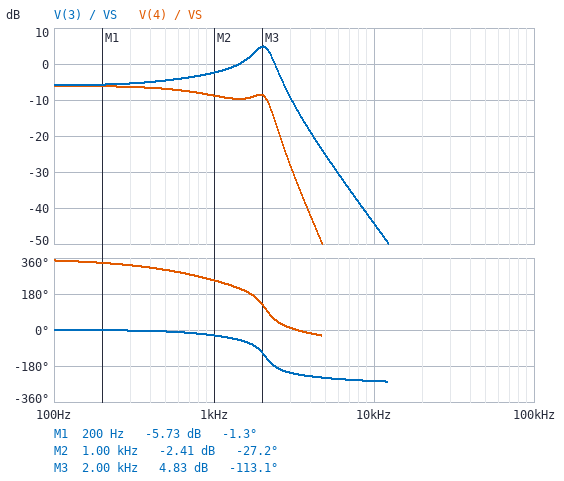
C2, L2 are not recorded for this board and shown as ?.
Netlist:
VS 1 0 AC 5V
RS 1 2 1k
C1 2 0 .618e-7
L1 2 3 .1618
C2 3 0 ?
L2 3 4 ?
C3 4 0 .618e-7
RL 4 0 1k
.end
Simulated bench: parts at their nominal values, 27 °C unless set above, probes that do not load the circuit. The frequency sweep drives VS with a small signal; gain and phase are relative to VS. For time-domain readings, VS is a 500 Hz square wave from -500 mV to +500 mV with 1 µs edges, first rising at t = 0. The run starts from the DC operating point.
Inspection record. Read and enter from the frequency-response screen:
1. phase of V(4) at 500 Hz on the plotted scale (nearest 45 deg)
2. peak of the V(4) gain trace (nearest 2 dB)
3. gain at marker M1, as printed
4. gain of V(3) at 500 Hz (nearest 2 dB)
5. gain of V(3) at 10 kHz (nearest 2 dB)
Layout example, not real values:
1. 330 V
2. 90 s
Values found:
1. 315 deg
2. -6 dB
3. -5.73 dB
4. -4 dB
5. -44 dB
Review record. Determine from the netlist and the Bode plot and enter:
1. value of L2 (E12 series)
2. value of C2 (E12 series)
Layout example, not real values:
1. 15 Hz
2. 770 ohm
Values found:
1. 330 mH
2. 68 nF
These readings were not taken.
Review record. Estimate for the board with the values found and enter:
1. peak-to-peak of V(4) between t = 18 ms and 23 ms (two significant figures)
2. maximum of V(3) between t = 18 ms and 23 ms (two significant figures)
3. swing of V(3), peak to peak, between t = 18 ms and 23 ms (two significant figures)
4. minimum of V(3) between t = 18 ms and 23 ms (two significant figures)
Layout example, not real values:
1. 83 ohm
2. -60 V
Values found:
1. 530 mV
2. 590 mV
3. 1.2 V
4. -590 mV
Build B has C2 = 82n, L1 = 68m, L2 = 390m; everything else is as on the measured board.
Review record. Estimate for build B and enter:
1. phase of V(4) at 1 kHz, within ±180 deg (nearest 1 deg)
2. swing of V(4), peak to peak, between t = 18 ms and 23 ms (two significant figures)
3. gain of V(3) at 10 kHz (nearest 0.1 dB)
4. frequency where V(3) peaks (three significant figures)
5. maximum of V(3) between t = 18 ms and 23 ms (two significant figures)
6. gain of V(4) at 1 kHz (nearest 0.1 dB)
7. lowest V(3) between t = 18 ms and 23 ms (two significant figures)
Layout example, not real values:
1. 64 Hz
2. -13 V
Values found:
1. -116 deg
2. 510 mV
3. -37.9 dB
4. 2.82 kHz
5. 630 mV
6. -9.5 dB
7. -630 mV
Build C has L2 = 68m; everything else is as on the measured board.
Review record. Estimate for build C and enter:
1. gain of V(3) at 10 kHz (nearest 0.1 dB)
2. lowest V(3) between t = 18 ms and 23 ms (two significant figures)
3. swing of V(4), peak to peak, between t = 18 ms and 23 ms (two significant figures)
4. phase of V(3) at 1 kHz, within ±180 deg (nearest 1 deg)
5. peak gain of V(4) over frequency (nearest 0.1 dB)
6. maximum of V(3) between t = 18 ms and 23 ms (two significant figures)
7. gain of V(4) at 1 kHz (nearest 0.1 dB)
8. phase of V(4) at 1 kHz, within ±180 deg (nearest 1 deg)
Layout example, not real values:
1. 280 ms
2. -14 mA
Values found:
1. -43.9 dB
2. -290 mV
3. 550 mV
4. -52 deg
5. -6.0 dB
6. 290 mV
7. -6.3 dB
8. -79 deg
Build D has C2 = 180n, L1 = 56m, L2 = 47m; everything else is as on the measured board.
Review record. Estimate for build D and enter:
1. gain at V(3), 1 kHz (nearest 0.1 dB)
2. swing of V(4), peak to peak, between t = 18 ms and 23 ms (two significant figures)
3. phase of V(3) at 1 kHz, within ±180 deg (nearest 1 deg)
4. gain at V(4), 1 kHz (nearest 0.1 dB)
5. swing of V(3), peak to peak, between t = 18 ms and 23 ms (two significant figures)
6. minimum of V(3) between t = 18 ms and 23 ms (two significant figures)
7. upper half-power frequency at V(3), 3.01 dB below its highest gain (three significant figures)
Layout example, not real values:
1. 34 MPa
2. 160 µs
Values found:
1. -7.6 dB
2. 560 mV
3. -49 deg
4. -7.0 dB
5. 510 mV
6. -250 mV
7. 3.46 kHz
